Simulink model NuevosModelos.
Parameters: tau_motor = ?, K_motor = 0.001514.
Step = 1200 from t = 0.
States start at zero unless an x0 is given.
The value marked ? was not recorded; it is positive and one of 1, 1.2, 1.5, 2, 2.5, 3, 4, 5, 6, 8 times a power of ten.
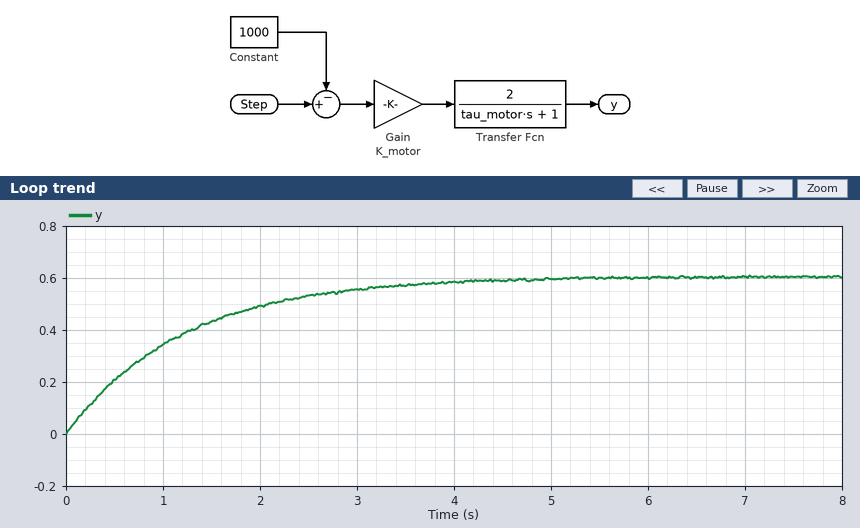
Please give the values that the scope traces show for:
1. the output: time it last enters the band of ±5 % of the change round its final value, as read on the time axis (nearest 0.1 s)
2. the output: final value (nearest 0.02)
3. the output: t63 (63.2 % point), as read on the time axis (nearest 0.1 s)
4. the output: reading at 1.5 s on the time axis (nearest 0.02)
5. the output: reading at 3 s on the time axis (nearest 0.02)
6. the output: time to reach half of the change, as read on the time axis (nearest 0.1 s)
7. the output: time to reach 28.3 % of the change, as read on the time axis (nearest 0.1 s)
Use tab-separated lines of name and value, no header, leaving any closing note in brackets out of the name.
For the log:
the output: time it last enters the band of ±5 % of the change round its final value, as read on the time axis	3.6 s
the output: final value	0.60
the output: t63 (63.2 % point), as read on the time axis	1.2 s
the output: reading at 1.5 s on the time axis	0.44
the output: reading at 3 s on the time axis	0.56
the output: time to reach half of the change, as read on the time axis	0.8 s
the output: time to reach 28.3 % of the change, as read on the time axis	0.4 s
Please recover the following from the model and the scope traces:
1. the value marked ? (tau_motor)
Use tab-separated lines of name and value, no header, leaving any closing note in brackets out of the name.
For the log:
the value marked ?	1.2
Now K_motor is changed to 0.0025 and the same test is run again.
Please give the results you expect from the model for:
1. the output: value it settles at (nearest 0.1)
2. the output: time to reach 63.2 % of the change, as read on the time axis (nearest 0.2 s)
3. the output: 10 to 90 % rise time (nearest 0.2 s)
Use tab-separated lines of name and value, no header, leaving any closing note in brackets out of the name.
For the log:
the output: value it settles at	1.0
the output: time to reach 63.2 % of the change, as read on the time axis	1.2 s
the output: 10 to 90 % rise time	2.6 s
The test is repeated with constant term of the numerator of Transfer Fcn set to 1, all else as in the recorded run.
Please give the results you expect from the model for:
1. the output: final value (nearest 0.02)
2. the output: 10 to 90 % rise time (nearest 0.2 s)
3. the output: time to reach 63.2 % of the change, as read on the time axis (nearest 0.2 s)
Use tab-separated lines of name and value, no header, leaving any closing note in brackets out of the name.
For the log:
the output: final value	0.30
the output: 10 to 90 % rise time	2.6 s
the output: time to reach 63.2 % of the change, as read on the time axis	1.2 s
